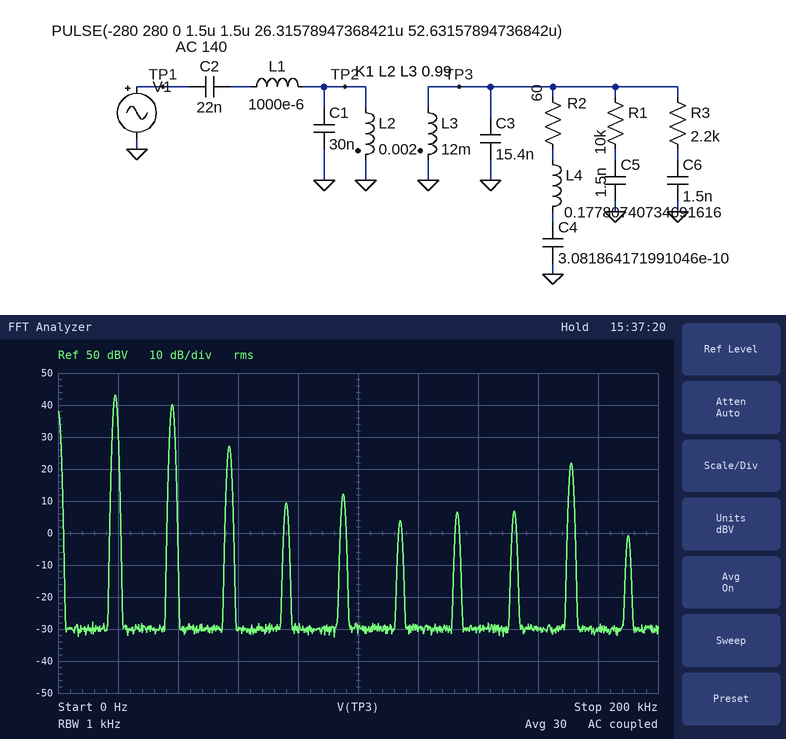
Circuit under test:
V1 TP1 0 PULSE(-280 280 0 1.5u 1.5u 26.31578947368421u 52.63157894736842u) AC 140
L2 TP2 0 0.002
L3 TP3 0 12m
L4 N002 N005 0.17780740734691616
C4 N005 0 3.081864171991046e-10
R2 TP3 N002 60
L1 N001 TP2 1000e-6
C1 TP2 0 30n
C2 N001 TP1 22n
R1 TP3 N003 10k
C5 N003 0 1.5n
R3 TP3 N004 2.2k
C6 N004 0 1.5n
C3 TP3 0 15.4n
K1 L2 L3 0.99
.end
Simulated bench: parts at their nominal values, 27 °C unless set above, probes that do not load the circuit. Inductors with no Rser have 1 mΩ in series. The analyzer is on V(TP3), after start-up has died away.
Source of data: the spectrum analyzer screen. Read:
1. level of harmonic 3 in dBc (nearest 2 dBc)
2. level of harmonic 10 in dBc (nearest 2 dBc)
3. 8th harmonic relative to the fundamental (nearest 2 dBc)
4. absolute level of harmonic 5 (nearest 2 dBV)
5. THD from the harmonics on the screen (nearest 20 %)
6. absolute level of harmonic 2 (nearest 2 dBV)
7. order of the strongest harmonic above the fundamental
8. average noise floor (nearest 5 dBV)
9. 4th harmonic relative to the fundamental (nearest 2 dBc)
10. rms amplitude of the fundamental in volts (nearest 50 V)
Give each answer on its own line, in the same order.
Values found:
-16 dBc
-44 dBc
-36 dBc
12 dBV
80 %
40 dBV
2
-30 dBV
-34 dBc
150 V
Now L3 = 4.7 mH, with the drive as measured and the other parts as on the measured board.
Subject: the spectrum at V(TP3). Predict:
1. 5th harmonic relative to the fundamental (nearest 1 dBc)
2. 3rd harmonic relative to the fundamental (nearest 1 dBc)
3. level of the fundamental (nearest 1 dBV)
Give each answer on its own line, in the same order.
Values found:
-32 dBc
-15 dBc
45 dBV
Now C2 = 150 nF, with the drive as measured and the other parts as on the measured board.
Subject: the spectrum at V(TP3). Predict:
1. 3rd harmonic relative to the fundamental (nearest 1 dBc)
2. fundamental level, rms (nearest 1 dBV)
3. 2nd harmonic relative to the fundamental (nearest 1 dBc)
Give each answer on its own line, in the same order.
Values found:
-48 dBc
72 dBV
-51 dBc
